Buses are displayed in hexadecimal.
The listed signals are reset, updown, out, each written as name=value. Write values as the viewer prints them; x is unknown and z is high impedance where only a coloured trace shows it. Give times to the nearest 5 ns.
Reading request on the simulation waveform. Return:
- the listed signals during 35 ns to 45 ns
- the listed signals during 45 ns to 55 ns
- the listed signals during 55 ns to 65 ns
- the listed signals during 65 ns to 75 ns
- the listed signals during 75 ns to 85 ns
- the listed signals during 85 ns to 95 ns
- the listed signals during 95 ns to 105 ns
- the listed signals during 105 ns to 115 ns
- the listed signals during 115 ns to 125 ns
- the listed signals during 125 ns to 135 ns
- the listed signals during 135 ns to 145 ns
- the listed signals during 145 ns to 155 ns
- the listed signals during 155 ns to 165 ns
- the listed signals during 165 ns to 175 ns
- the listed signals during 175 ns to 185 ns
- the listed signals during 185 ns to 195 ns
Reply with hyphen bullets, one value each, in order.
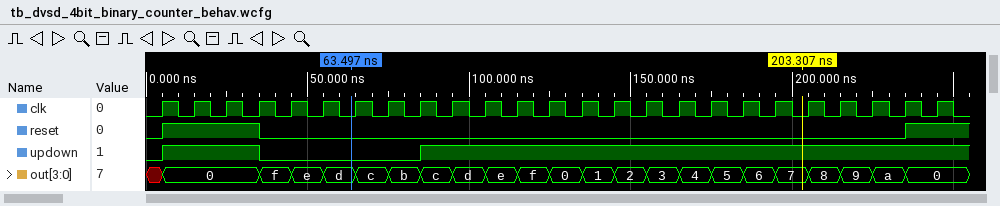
- reset=0, updown=0, out=f
- reset=0, updown=0, out=e
- reset=0, updown=0, out=d
- reset=0, updown=0, out=c
- reset=0, updown=0, out=b
- reset=0, updown=1, out=c
- reset=0, updown=1, out=d
- reset=0, updown=1, out=e
- reset=0, updown=1, out=f
- reset=0, updown=1, out=0
- reset=0, updown=1, out=1
- reset=0, updown=1, out=2
- reset=0, updown=1, out=3
- reset=0, updown=1, out=4
- reset=0, updown=1, out=5
- reset=0, updown=1, out=6
